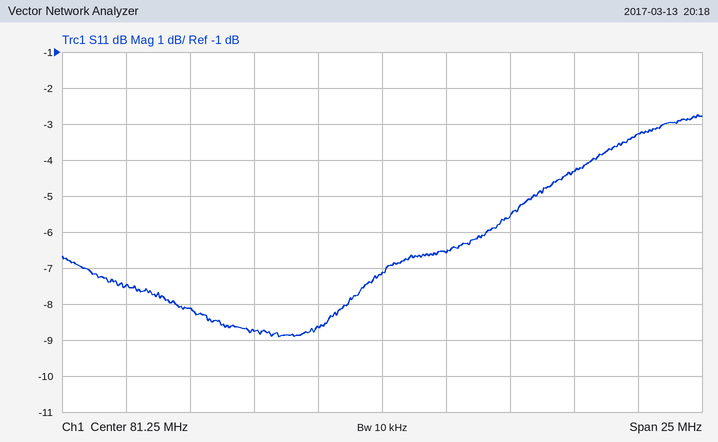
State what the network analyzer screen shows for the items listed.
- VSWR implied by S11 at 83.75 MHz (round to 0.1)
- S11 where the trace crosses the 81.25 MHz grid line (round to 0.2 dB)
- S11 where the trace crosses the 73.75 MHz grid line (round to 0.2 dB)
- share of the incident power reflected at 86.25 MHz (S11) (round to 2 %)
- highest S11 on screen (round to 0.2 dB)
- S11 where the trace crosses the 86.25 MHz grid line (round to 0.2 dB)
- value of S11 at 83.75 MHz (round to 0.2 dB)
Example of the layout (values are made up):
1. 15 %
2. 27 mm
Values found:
1. 2.8
2. -7.2 dB
3. -8.2 dB
4. 28 %
5. -2.8 dB
6. -5.6 dB
7. -6.6 dB
